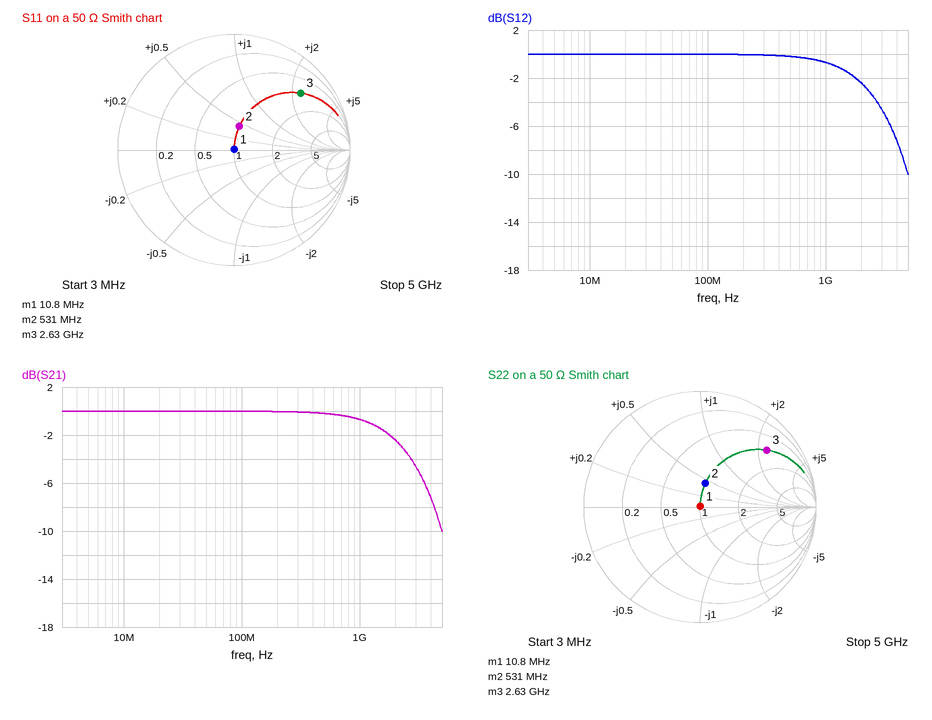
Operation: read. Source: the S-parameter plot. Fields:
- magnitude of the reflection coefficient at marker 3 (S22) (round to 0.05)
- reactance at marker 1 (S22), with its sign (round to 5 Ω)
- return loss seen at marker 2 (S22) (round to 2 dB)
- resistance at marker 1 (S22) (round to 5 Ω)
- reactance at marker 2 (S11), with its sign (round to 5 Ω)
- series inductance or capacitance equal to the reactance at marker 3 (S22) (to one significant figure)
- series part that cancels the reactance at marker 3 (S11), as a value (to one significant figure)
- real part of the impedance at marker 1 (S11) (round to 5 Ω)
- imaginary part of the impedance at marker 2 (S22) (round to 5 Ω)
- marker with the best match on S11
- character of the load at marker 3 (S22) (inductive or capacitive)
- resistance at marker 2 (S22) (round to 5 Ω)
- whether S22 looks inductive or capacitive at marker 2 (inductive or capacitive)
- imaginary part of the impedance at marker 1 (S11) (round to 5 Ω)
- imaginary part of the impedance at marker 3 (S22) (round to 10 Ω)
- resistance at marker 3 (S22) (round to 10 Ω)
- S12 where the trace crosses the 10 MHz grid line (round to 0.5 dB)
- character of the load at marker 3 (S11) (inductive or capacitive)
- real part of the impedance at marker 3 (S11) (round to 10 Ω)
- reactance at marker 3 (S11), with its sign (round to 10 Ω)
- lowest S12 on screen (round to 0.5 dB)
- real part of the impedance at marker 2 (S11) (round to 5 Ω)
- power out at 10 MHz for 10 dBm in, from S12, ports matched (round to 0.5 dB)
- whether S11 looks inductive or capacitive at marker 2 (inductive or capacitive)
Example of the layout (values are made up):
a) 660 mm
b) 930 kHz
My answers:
a) 0.75
b) 0 Ω
c) 14 dB
d) 50 Ω
e) +20 Ω
f) 7 nH
g) 500 fF
h) 50 Ω
i) +20 Ω
j) marker 1
k) inductive
l) 50 Ω
m) inductive
n) 0 Ω
o) +120 Ω
p) 50 Ω
q) 0.0 dB
r) inductive
s) 50 Ω
t) +120 Ω
u) -10.0 dB
v) 50 Ω
w) 10.0 dBm
x) inductive
